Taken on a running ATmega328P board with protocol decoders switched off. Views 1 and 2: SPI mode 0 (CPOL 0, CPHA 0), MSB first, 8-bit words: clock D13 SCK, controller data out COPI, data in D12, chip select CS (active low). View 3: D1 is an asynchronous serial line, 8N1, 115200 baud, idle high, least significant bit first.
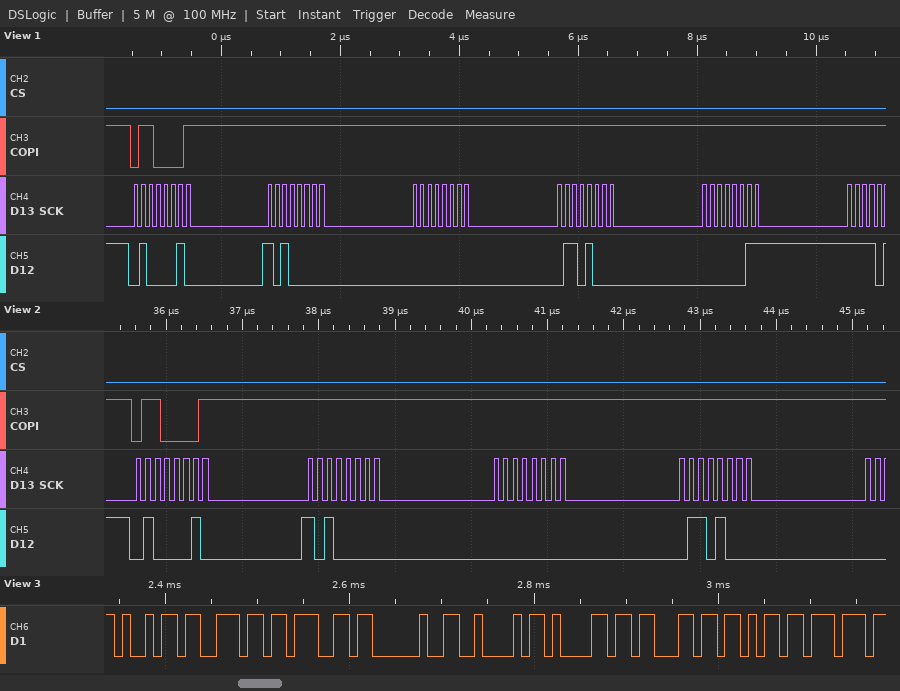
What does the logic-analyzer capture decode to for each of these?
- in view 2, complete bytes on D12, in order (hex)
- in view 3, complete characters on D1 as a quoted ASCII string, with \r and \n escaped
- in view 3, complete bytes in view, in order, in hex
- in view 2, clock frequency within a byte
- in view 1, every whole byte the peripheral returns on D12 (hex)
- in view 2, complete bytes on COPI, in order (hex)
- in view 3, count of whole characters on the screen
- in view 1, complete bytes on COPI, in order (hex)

42 A0 00 68
"ing Backw"
69 6E 67 20 42 61 63 6B 77
8 MHz
42 A0 00 68 03
61 FF FF FF
9
61 FF FF FF FF
